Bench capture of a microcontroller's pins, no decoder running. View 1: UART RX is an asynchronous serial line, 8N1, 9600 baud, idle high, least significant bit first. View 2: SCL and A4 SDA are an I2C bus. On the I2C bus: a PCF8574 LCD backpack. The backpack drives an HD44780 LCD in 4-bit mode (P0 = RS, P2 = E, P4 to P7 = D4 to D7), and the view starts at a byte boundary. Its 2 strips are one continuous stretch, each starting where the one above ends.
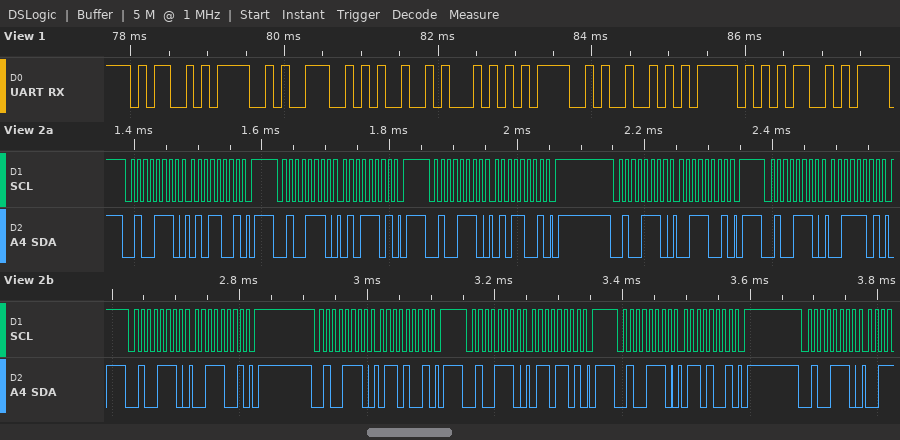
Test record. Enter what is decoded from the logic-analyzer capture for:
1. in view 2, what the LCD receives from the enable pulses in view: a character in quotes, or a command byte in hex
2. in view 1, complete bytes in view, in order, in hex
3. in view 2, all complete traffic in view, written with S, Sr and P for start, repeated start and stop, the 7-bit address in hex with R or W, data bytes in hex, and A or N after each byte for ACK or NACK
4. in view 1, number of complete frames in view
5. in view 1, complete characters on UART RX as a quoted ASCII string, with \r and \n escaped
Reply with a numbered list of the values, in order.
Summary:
1. 'S'
2. 4D 4F 4E 49 54 4F 52 5F 4D
3. S 27W A 59 A P S 27W A 5D A P S 27W A 59 A P S 27W A 39 A P S 27W A 3D A P S 27W A 39 A P S 27W A 69 A P S 27W A 6D A P S 27W A 69 A P S 27W A
4. 9
5. "MONITOR_M"
